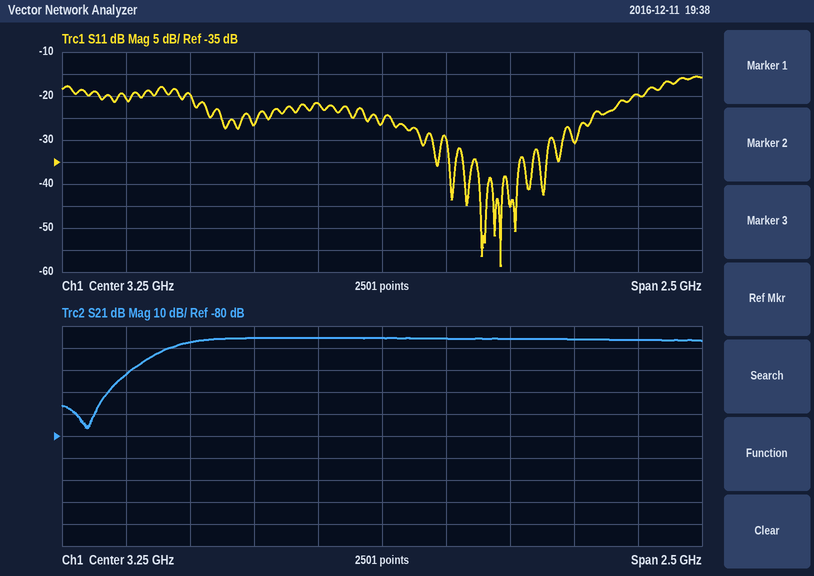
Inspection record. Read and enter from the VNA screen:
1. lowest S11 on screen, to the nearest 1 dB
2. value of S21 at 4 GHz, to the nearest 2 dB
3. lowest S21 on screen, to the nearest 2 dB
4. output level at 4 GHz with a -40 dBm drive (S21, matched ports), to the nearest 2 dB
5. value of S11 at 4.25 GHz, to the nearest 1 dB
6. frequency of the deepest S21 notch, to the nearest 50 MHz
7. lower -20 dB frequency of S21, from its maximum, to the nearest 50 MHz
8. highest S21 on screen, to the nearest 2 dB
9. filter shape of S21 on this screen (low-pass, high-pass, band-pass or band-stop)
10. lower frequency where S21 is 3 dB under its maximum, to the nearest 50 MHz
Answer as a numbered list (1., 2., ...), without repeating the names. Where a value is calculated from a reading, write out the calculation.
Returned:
1. -59 dB
2. -36 dB
3. -76 dB
4. -40 dBm + (-36 dB) = -76 dBm
5. -20 dB
6. 2.10 GHz
7. 2.20 GHz
8. -36 dB
9. high-pass
10. 2.45 GHz
